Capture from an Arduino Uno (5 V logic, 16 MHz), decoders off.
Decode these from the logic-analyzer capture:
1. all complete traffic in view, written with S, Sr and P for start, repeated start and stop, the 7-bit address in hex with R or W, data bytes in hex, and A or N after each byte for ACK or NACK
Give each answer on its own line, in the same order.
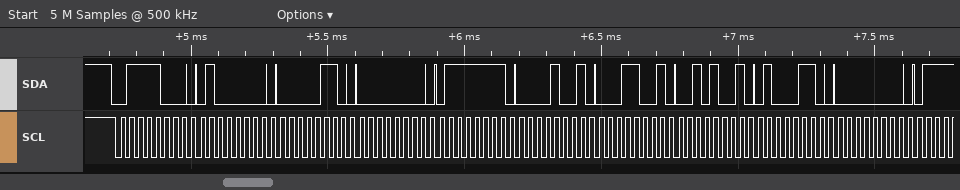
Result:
S 3CW A 40 A 06 A 00 A 7F A 09 A 19 A 29 A 46 A 00 A
